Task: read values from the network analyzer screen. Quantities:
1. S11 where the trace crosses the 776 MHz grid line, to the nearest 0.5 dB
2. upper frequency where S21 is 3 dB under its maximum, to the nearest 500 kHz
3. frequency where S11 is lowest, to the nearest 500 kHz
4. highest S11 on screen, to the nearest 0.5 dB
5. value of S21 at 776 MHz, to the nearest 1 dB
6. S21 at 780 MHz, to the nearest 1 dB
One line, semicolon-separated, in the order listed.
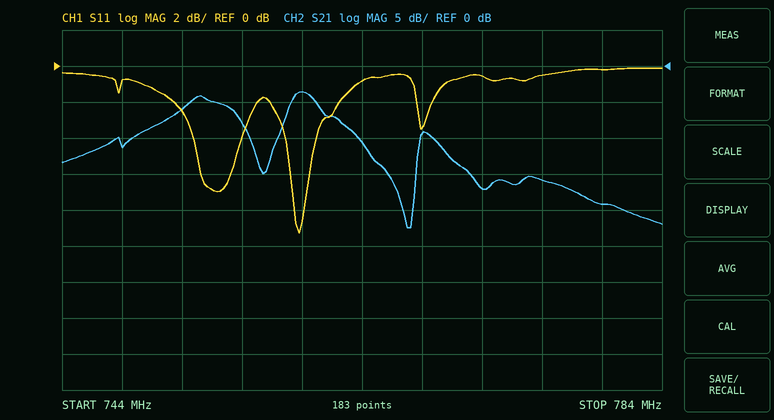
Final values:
-0.5 dB; 761.5 MHz; 760.0 MHz; 0.0 dB; -16 dB; -19 dB
